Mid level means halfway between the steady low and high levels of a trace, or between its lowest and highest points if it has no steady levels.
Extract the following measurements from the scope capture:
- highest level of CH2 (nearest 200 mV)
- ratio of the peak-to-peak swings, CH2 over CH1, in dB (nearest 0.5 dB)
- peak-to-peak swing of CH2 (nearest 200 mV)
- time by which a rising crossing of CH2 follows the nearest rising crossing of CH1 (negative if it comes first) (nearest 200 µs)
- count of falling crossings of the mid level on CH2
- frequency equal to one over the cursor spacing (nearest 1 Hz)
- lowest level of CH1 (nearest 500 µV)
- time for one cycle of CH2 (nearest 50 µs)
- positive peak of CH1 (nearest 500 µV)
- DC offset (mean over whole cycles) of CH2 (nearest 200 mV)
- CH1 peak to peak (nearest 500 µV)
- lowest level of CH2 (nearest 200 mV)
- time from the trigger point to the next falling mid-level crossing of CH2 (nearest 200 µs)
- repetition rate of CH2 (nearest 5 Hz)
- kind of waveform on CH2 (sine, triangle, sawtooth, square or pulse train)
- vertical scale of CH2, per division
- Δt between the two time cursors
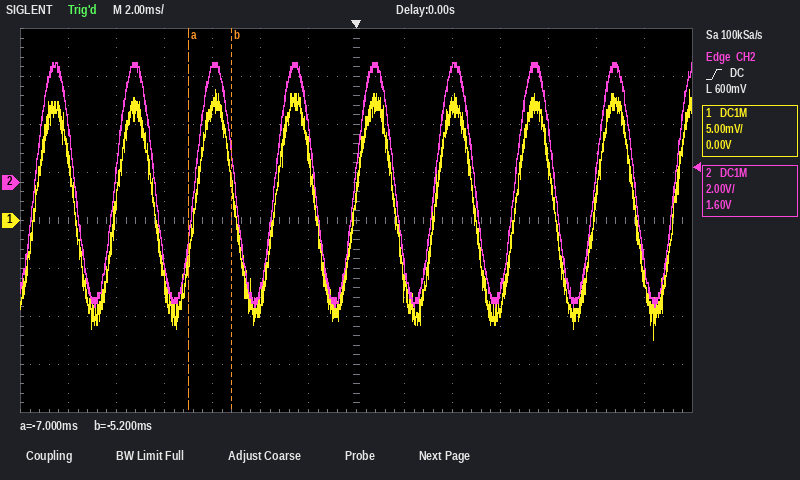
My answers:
5.0 V
52.0 dB
10.2 V
0.0 ms
8
556 Hz
-12.5 mV
3.35 ms
13.5 mV
0.0 V
26.0 mV
-5.2 V
1.6 ms
300 Hz
sine
2 V
1.8 ms
